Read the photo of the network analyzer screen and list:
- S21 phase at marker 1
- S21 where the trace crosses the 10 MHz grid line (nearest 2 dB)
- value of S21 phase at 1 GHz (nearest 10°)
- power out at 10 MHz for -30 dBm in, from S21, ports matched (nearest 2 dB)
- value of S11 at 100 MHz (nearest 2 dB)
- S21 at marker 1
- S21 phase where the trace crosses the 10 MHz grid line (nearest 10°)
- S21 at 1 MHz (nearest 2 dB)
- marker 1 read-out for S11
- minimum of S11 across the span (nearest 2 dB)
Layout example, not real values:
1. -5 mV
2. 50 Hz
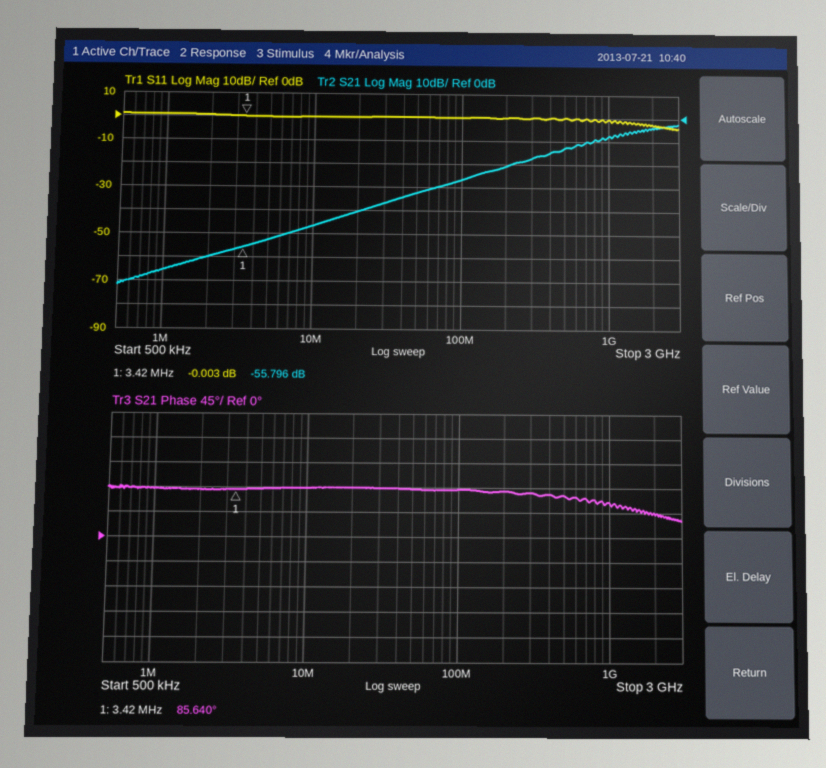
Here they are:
1. 85.640°
2. -46 dB
3. 60°
4. -76 dBm
5. 0 dB
6. -55.796 dB
7. 90°
8. -66 dB
9. -0.003 dB
10. -4 dB
